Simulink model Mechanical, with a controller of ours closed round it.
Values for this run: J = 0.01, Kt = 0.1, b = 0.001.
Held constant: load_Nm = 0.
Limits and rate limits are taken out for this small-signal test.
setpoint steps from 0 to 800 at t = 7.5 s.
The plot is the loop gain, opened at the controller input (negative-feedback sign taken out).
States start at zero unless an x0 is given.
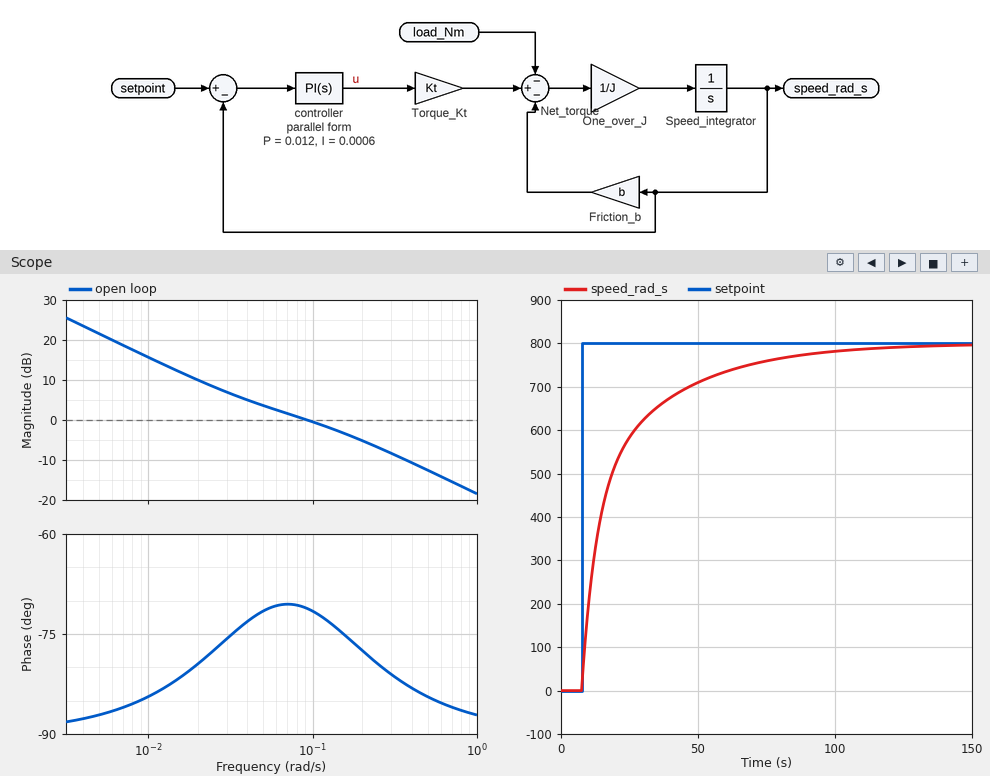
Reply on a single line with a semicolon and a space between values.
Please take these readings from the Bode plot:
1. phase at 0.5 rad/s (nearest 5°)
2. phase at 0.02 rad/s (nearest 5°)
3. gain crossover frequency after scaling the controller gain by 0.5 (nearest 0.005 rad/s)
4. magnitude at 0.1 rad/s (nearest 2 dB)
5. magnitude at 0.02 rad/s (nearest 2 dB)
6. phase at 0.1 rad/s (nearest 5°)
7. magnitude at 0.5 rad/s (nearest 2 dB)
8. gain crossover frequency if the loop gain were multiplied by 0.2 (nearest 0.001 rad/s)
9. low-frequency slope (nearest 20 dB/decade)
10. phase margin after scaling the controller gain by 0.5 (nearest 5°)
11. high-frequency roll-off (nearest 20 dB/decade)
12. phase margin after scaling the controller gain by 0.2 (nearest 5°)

-85°; -80°; 0.035 rad/s; 0 dB; 10 dB; -70°; -12 dB; 0.012 rad/s; -20 dB/decade; 105°; -20 dB/decade; 95°
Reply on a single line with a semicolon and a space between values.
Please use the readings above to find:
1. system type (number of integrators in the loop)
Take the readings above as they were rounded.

1
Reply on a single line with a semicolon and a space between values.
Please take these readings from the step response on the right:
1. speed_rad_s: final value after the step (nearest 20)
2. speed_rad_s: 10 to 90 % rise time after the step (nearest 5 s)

800; 45 s
